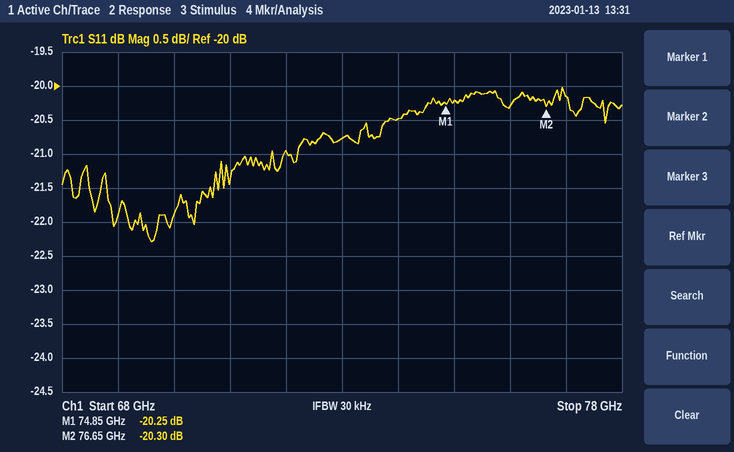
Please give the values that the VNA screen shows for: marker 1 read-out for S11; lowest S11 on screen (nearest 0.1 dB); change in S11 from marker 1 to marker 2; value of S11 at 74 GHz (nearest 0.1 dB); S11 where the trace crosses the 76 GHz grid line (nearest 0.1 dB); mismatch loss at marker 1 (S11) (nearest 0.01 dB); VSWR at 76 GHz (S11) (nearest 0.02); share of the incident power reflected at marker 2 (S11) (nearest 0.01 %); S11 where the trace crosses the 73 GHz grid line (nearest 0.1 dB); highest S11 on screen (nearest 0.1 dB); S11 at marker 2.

-20.25 dB
-22.3 dB
-0.05 dB
-20.5 dB
-20.3 dB
0.04 dB
1.22
0.93 %
-20.8 dB
-20.0 dB
-20.30 dB
